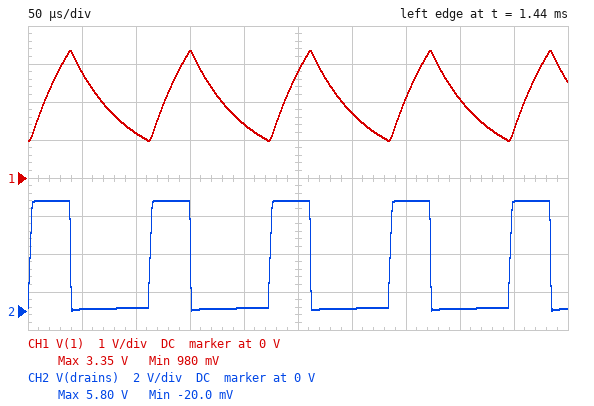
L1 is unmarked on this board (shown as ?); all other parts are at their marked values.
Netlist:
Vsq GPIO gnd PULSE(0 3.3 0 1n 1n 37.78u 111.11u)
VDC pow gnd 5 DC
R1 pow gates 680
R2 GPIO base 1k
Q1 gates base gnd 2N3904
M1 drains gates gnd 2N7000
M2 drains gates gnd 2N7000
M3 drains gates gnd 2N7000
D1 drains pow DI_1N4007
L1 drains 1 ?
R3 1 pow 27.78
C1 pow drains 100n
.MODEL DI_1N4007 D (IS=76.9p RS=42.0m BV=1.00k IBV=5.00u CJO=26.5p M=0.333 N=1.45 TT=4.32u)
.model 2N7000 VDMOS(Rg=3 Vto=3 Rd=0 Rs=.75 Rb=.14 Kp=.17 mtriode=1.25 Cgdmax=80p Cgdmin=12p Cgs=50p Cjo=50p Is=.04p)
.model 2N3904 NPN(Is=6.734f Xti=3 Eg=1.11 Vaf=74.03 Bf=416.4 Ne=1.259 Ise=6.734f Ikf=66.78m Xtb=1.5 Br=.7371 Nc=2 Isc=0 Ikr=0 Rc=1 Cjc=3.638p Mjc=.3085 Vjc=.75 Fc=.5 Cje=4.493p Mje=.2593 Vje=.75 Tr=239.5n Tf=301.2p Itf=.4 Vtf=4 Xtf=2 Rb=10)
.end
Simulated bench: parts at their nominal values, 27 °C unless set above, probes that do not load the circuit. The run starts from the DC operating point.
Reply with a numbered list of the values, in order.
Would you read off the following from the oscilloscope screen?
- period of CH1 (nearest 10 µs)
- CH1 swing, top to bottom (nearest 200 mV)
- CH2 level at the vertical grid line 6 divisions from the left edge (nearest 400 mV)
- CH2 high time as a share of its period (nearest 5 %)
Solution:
1. 110 µs
2. 2.4 V
3. 0 V
4. 35 %
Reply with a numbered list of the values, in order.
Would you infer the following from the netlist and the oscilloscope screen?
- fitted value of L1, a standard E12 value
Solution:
1. 1.5 mH
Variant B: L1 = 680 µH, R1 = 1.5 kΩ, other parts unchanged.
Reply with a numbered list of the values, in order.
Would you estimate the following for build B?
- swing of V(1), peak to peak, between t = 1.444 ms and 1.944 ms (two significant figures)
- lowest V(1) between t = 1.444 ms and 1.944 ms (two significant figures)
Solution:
1. 4.2 V
2. 400 mV
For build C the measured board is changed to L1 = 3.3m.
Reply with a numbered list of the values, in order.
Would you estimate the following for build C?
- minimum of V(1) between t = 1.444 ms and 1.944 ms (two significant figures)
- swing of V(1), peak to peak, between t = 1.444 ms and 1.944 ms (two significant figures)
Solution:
1. 1.5 V
2. 1.1 V
